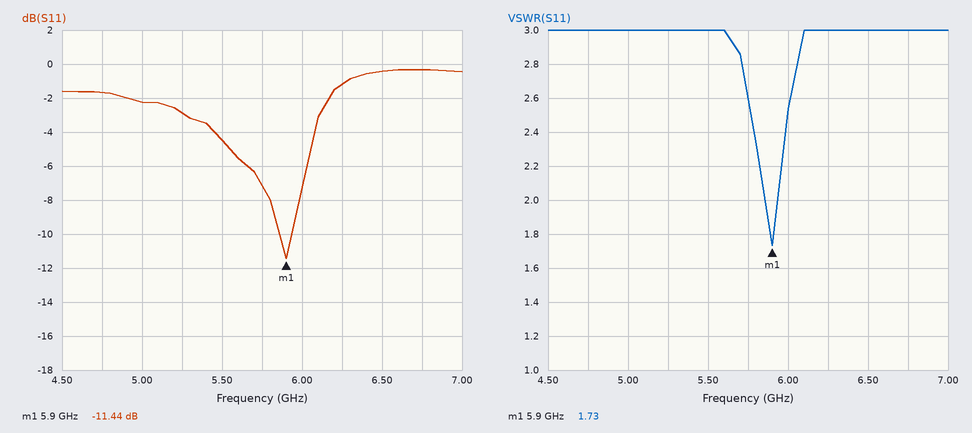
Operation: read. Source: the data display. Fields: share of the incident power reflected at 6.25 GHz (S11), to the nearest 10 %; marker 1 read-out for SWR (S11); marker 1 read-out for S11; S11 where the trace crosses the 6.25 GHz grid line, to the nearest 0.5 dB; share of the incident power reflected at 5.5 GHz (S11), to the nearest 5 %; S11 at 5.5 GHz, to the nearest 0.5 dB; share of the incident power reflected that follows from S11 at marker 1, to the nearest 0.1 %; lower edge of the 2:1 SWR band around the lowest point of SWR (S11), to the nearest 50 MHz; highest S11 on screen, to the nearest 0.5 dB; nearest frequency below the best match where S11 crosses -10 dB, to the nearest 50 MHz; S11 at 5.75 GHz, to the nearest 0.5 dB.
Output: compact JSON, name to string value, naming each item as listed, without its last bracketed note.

{"share of the incident power reflected at 6.25 GHz (S11), to the nearest 10 %": "80 %", "marker 1 read-out for SWR": "1.73", "marker 1 read-out for S11": "-11.44 dB", "S11 where the trace crosses the 6.25 GHz grid line, to the nearest 0.5 dB": "-1.0 dB", "share of the incident power reflected at 5.5 GHz (S11), to the nearest 5 %": "35 %", "S11 at 5.5 GHz, to the nearest 0.5 dB": "-4.5 dB", "share of the incident power reflected that follows from S11 at marker 1, to the nearest 0.1 %": "7.2 %", "lower edge of the 2:1 SWR band around the lowest point of SWR (S11), to the nearest 50 MHz": "5.85 GHz", "highest S11 on screen, to the nearest 0.5 dB": "-0.5 dB", "nearest frequency below the best match where S11 crosses -10 dB, to the nearest 50 MHz": "5.85 GHz", "S11 at 5.75 GHz, to the nearest 0.5 dB": "-7.0 dB"}
